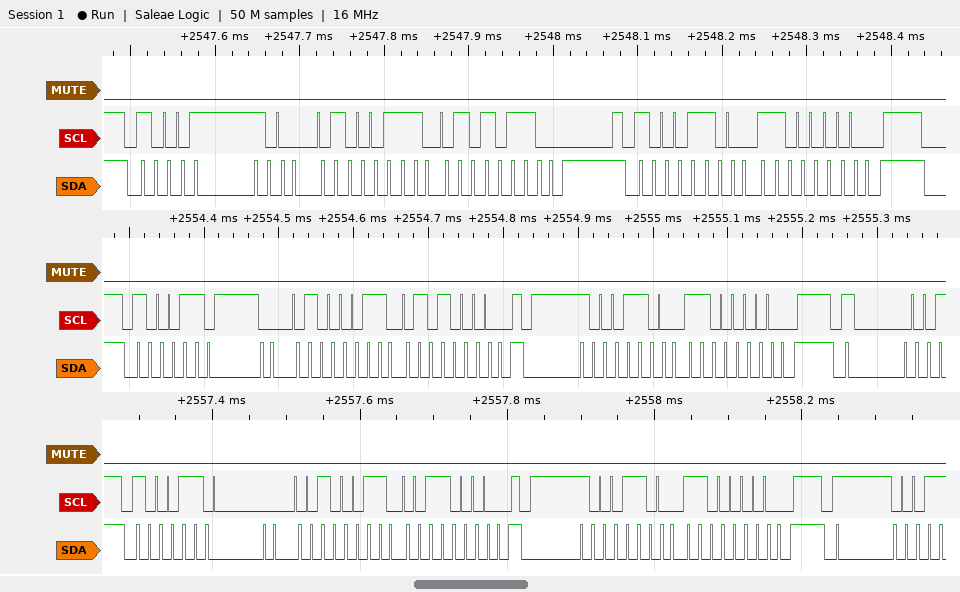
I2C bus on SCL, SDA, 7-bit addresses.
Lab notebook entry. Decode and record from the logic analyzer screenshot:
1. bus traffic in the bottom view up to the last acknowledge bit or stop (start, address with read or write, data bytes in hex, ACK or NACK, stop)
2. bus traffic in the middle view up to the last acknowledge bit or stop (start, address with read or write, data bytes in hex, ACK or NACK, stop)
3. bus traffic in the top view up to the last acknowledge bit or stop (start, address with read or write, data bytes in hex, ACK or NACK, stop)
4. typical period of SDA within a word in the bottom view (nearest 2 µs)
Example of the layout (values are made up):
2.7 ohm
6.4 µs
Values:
start, address 46 write ACK, 23 ACK, 30 ACK, stop, start, address 46 write ACK, C0 ACK, stop
start, address 46 write ACK, 43 ACK, 50 ACK, stop, start, address 46 write ACK, C0 ACK, stop
start, address 46 write ACK, 47 ACK, 56 ACK, stop, start, address 46 write ACK, C0 ACK, stop
16 µs
